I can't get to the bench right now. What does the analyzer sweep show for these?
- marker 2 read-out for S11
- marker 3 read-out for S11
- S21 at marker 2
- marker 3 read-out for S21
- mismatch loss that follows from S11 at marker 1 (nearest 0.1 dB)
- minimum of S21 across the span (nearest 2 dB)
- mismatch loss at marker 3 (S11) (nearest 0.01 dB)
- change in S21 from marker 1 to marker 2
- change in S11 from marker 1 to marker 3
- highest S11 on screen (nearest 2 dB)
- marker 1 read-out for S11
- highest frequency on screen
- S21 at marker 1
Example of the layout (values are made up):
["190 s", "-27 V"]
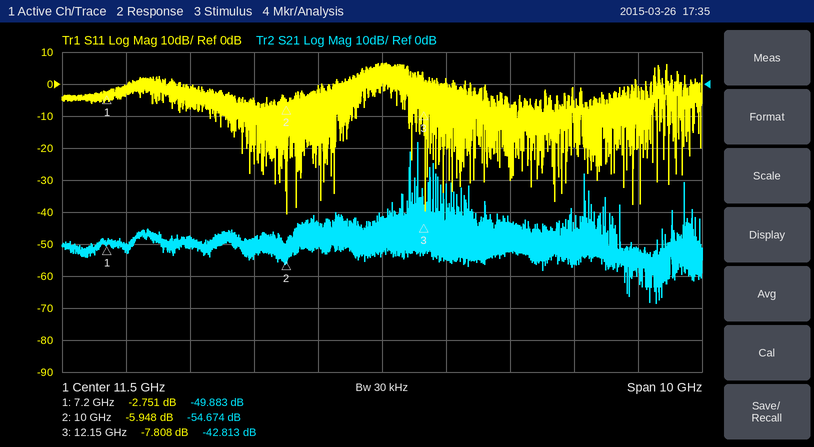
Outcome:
["-5.948 dB", "-7.808 dB", "-54.674 dB", "-42.813 dB", "3.3 dB", "-68 dB", "0.79 dB", "-4.791 dB", "-5.057 dB", "6 dB", "-2.751 dB", "16.5 GHz", "-49.883 dB"]
